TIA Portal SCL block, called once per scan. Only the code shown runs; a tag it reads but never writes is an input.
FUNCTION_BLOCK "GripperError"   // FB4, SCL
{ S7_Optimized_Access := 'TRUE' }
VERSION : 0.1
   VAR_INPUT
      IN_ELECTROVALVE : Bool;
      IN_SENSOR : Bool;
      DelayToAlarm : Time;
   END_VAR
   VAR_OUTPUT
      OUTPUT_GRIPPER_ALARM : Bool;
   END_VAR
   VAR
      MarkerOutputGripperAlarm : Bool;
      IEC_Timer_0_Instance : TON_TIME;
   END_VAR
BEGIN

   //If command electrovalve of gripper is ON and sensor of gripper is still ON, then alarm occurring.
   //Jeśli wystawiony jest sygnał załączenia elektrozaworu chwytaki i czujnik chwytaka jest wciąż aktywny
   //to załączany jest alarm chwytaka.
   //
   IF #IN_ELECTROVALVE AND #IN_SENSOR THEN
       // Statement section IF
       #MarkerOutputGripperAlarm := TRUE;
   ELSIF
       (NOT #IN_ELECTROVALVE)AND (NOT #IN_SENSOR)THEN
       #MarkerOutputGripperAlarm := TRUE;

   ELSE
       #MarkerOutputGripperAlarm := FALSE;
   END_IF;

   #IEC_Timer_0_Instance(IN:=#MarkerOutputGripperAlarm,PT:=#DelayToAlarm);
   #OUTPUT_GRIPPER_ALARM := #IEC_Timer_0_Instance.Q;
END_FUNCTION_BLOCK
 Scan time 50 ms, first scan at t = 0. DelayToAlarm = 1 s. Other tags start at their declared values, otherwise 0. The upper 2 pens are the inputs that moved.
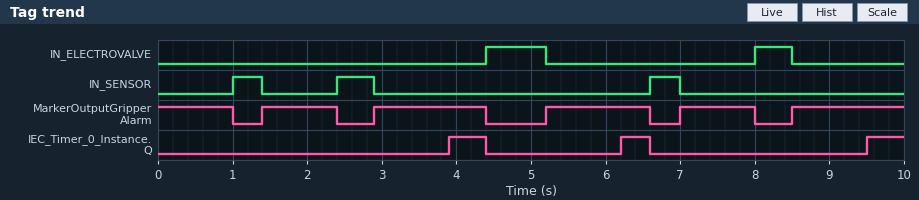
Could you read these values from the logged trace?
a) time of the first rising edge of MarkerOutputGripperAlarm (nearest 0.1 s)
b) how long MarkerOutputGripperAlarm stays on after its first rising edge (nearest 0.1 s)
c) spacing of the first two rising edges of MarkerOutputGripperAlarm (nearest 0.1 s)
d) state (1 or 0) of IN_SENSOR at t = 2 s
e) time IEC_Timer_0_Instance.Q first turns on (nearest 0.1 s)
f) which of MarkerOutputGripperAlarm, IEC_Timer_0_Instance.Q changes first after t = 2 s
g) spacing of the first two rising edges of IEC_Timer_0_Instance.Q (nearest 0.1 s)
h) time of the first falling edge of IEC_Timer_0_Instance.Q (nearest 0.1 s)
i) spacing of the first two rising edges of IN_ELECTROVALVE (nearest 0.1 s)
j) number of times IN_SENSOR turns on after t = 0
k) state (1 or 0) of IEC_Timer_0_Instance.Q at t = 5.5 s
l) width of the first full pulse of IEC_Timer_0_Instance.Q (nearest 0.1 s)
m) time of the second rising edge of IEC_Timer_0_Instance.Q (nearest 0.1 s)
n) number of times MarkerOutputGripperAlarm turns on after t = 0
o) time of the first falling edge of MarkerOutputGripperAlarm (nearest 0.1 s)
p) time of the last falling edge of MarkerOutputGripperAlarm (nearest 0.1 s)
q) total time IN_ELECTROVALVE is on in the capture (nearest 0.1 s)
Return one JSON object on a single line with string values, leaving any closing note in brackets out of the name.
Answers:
{"time of the first rising edge of MarkerOutputGripperAlarm": "1.4 s", "how long MarkerOutputGripperAlarm stays on after its first rising edge": "1.0 s", "spacing of the first two rising edges of MarkerOutputGripperAlarm": "1.5 s", "state (1 or 0) of IN_SENSOR at t = 2 s": "0", "time IEC_Timer_0_Instance.Q first turns on": "3.9 s", "which of MarkerOutputGripperAlarm, IEC_Timer_0_Instance.Q changes first after t = 2 s": "MarkerOutputGripperAlarm", "spacing of the first two rising edges of IEC_Timer_0_Instance.Q": "2.3 s", "time of the first falling edge of IEC_Timer_0_Instance.Q": "4.4 s", "spacing of the first two rising edges of IN_ELECTROVALVE": "3.6 s", "number of times IN_SENSOR turns on after t = 0": "3", "state (1 or 0) of IEC_Timer_0_Instance.Q at t = 5.5 s": "0", "width of the first full pulse of IEC_Timer_0_Instance.Q": "0.5 s", "time of the second rising edge of IEC_Timer_0_Instance.Q": "6.2 s", "number of times MarkerOutputGripperAlarm turns on after t = 0": "5", "time of the first falling edge of MarkerOutputGripperAlarm": "1.0 s", "time of the last falling edge of MarkerOutputGripperAlarm": "8.0 s", "total time IN_ELECTROVALVE is on in the capture": "1.3 s"}
